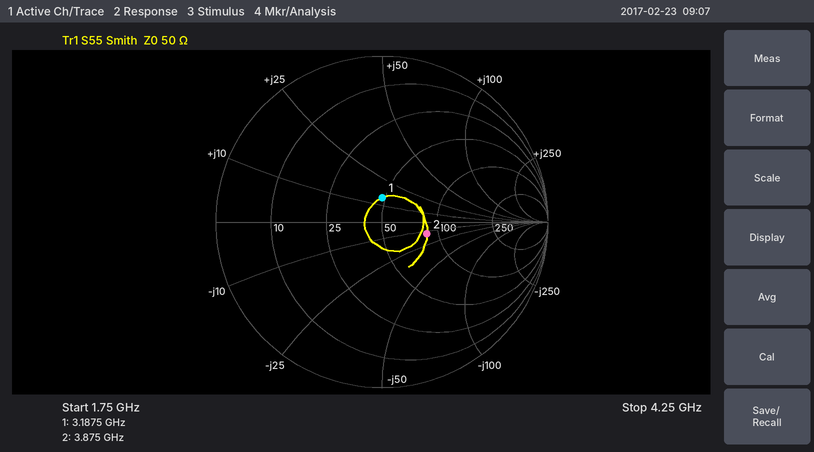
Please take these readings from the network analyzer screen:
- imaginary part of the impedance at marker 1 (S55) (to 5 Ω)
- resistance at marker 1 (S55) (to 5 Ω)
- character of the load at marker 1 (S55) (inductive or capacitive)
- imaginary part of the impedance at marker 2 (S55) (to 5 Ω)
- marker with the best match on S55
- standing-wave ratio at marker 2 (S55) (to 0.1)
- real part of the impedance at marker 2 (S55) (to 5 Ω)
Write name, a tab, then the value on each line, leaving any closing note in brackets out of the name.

imaginary part of the impedance at marker 1 (S55)	+15 Ω
resistance at marker 1 (S55)	50 Ω
character of the load at marker 1 (S55)	inductive
imaginary part of the impedance at marker 2 (S55)	-15 Ω
marker with the best match on S55	marker 1
standing-wave ratio at marker 2 (S55)	1.8
real part of the impedance at marker 2 (S55)	85 Ω
